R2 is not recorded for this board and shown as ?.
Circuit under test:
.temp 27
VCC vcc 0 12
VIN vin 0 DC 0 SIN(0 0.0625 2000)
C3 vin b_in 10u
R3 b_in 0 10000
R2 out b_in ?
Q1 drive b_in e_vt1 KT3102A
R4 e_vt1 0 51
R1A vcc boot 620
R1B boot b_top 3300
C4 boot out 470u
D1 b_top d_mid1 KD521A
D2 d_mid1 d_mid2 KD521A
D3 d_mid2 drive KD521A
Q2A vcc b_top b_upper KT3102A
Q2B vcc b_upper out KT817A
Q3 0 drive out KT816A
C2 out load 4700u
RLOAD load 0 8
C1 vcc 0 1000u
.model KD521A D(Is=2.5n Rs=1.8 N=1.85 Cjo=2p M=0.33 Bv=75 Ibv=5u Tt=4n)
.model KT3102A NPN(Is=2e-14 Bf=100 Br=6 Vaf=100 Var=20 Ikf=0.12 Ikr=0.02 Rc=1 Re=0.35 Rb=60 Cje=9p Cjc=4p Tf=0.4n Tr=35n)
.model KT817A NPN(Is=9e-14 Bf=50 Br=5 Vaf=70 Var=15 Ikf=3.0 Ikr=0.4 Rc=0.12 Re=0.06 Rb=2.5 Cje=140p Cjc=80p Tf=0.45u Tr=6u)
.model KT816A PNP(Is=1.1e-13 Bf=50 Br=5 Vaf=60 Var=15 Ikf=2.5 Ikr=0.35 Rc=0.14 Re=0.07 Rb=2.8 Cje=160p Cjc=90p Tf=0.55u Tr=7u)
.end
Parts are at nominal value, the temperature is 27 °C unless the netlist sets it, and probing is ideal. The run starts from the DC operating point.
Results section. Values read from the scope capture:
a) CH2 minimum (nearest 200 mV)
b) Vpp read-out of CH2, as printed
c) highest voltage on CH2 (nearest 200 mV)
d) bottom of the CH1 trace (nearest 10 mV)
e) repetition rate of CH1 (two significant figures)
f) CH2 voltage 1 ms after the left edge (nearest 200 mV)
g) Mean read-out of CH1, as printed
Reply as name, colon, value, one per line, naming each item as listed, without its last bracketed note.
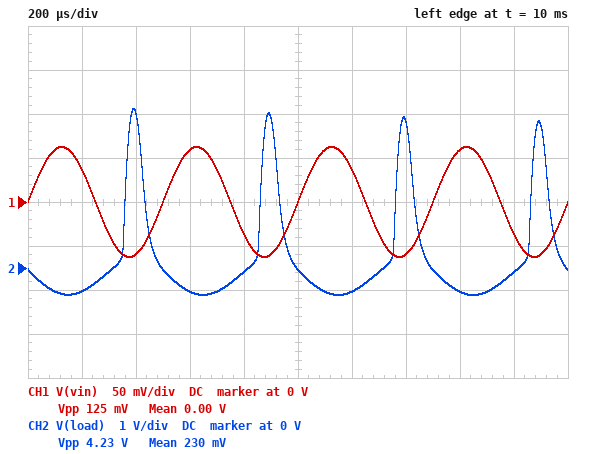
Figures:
CH2 minimum: -600 mV
Vpp read-out of CH2, as printed: 4.23 V
highest voltage on CH2: 3.6 V
bottom of the CH1 trace: -60 mV
repetition rate of CH1: 2.0 kHz
CH2 voltage 1 ms after the left edge: 0 V
Mean read-out of CH1, as printed: 0.00 V
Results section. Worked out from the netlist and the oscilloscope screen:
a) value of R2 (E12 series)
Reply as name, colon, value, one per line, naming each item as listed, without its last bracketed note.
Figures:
value of R2: 33 kΩ
